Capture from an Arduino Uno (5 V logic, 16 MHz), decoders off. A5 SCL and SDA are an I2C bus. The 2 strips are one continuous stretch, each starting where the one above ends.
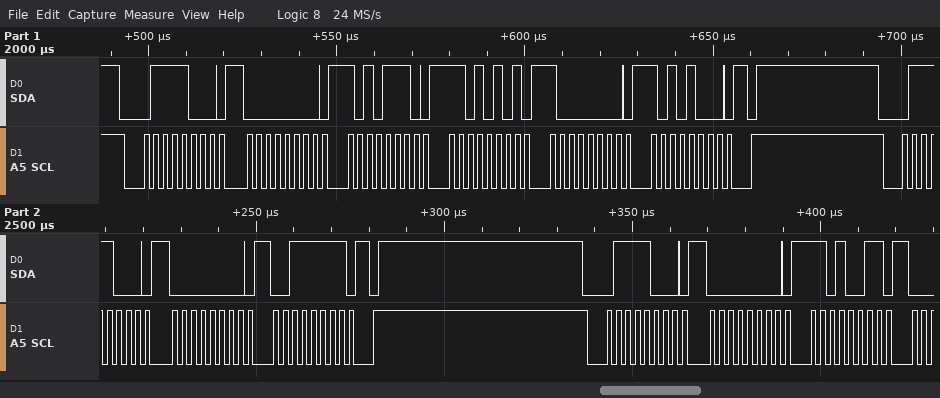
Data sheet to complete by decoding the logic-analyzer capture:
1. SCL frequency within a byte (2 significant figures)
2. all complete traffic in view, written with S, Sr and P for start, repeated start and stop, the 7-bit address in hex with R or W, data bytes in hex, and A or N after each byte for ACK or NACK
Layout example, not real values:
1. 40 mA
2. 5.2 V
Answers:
1. 400 kHz
2. S 3CW A 00 A AE A D5 A 80 A A8 A P S 3CW A 00 A 3F A P S 3CW A 00 A D3 A
